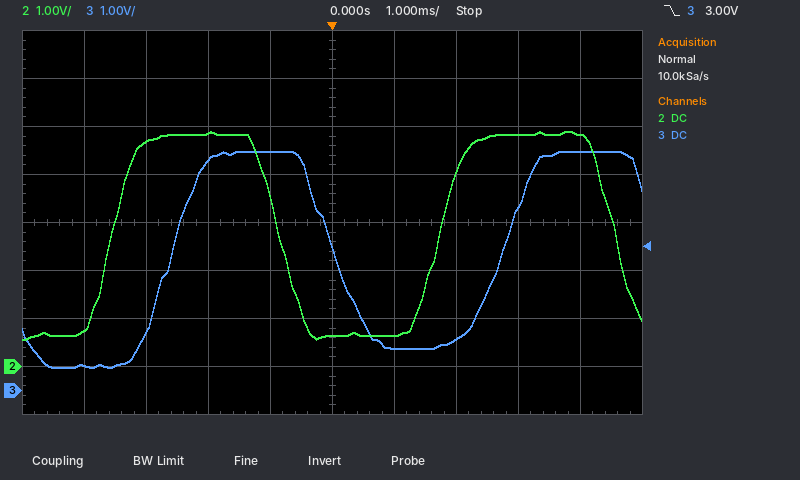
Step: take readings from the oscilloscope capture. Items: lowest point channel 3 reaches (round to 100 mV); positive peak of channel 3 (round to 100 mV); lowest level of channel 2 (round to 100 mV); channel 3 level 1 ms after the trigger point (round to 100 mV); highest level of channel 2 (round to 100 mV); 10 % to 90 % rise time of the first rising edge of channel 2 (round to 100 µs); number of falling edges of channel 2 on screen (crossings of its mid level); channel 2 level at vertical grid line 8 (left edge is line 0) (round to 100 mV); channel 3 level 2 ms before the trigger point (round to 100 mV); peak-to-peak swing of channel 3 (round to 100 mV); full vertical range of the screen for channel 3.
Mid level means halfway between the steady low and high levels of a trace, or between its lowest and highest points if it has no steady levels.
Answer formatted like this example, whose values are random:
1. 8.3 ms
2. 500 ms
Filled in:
1. 500 mV
2. 5.0 V
3. 600 mV
4. 900 mV
5. 4.9 V
6. 700 µs
7. 2
8. 4.8 V
9. 4.8 V
10. 4.5 V
11. 8 V
